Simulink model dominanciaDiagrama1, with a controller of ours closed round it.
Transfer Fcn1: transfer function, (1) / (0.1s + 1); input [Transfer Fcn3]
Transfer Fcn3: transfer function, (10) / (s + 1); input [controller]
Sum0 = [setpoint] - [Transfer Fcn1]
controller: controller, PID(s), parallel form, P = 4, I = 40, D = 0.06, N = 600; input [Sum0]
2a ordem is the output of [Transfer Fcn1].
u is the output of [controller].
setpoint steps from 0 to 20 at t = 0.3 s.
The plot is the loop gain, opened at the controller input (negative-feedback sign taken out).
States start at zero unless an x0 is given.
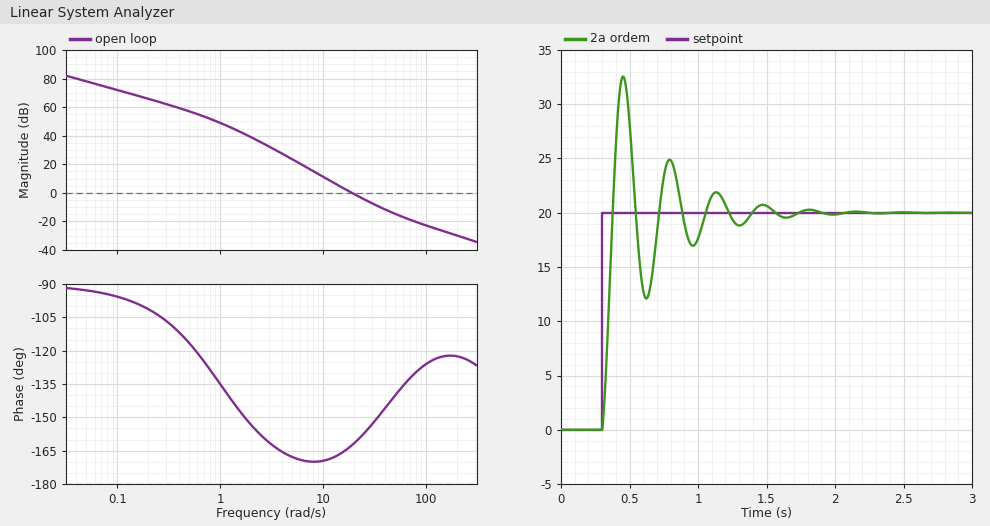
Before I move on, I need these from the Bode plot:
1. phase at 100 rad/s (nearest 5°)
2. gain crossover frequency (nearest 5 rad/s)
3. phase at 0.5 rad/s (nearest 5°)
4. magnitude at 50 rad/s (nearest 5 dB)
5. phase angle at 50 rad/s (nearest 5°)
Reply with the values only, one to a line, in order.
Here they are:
-125°
20 rad/s
-115°
-15 dB
-140°
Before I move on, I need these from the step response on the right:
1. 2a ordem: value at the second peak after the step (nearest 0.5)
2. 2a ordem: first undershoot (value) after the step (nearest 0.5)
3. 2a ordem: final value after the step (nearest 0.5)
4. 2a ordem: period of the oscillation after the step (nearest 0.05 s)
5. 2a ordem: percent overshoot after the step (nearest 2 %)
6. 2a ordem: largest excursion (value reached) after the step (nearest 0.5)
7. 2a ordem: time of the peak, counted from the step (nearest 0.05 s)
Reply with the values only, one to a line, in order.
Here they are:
25.0
12.0
20.0
0.35 s
62 %
32.5
0.15 s
